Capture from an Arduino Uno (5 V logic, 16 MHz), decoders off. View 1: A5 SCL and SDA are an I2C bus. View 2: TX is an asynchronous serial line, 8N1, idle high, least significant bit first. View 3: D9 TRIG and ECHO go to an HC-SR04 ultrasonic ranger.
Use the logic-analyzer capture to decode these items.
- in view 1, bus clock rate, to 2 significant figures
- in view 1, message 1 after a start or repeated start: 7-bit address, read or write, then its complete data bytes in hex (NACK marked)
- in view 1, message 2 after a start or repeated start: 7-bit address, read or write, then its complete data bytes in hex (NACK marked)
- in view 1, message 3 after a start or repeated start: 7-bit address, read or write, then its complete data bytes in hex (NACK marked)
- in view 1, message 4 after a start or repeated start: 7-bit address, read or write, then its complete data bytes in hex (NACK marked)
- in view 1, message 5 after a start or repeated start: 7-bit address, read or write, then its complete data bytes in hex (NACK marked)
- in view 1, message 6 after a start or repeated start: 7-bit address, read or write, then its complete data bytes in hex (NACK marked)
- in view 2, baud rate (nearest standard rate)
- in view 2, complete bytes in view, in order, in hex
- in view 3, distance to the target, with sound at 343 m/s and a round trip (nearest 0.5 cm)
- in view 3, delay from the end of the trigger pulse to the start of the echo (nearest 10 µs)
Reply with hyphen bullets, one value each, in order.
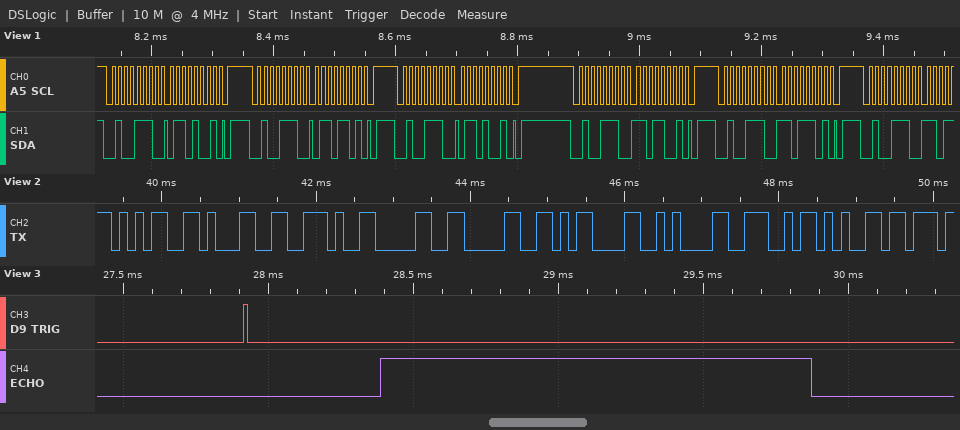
- 100 kHz
- 0x27 write: 69
- 0x27 write: 6D
- 0x27 write: 69
- 0x27 write: D9
- 0x27 write: DD
- 0x27 write
- 9600 baud
- 35 31 2E 30 30 0D 0A 4E 65
- 25.5 cm
- 460 µs
